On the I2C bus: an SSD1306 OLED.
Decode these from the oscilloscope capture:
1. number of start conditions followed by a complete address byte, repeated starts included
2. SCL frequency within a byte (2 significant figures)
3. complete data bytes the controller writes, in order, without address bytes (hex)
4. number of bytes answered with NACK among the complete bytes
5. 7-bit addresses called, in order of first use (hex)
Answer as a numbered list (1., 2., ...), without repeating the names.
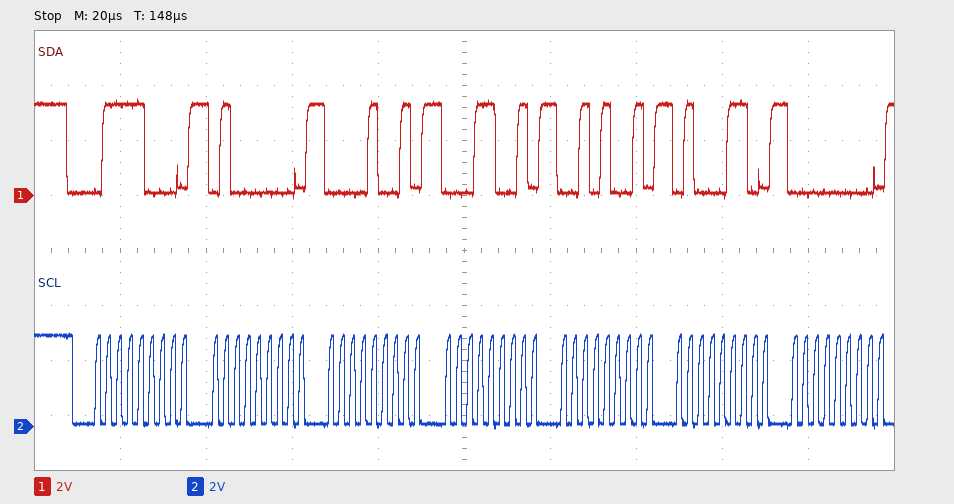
1. 1
2. 400 kHz
3. 40 09 19 29 46 00
4. 0
5. 0x3C
